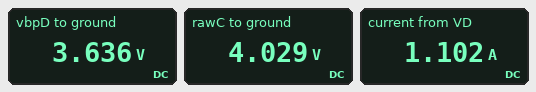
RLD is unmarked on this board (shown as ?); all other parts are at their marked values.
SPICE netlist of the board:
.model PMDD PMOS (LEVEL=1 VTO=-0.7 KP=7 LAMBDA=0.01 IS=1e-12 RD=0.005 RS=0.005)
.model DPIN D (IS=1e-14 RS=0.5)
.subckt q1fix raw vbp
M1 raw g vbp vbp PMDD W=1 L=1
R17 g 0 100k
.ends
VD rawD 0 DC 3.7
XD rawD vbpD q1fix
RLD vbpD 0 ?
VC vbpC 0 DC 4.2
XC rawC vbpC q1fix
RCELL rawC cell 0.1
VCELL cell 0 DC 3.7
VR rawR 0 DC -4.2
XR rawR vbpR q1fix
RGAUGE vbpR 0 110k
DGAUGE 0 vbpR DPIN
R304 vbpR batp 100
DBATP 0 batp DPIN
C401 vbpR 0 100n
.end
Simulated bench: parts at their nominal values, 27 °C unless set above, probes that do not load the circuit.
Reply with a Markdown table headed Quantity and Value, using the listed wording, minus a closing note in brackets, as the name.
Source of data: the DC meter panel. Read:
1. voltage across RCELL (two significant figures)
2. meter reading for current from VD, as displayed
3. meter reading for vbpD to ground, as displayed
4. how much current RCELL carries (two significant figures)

| Quantity | Value |
|---|---|
| voltage across RCELL | 330 mV |
| meter reading for current from VD, as displayed | 1.102 A |
| meter reading for vbpD to ground, as displayed | 3.636 V |
| how much current RCELL carries | 3.3 A |
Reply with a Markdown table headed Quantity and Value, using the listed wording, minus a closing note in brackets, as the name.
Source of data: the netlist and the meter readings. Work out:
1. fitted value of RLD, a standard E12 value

| Quantity | Value |
|---|---|
| fitted value of RLD, a standard E12 value | 3.3 Ω |
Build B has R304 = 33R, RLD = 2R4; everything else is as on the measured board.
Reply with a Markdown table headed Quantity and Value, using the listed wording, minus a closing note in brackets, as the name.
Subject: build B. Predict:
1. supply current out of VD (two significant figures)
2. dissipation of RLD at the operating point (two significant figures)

| Quantity | Value |
|---|---|
| supply current out of VD | 1.5 A |
| dissipation of RLD at the operating point | 5.4 W |
